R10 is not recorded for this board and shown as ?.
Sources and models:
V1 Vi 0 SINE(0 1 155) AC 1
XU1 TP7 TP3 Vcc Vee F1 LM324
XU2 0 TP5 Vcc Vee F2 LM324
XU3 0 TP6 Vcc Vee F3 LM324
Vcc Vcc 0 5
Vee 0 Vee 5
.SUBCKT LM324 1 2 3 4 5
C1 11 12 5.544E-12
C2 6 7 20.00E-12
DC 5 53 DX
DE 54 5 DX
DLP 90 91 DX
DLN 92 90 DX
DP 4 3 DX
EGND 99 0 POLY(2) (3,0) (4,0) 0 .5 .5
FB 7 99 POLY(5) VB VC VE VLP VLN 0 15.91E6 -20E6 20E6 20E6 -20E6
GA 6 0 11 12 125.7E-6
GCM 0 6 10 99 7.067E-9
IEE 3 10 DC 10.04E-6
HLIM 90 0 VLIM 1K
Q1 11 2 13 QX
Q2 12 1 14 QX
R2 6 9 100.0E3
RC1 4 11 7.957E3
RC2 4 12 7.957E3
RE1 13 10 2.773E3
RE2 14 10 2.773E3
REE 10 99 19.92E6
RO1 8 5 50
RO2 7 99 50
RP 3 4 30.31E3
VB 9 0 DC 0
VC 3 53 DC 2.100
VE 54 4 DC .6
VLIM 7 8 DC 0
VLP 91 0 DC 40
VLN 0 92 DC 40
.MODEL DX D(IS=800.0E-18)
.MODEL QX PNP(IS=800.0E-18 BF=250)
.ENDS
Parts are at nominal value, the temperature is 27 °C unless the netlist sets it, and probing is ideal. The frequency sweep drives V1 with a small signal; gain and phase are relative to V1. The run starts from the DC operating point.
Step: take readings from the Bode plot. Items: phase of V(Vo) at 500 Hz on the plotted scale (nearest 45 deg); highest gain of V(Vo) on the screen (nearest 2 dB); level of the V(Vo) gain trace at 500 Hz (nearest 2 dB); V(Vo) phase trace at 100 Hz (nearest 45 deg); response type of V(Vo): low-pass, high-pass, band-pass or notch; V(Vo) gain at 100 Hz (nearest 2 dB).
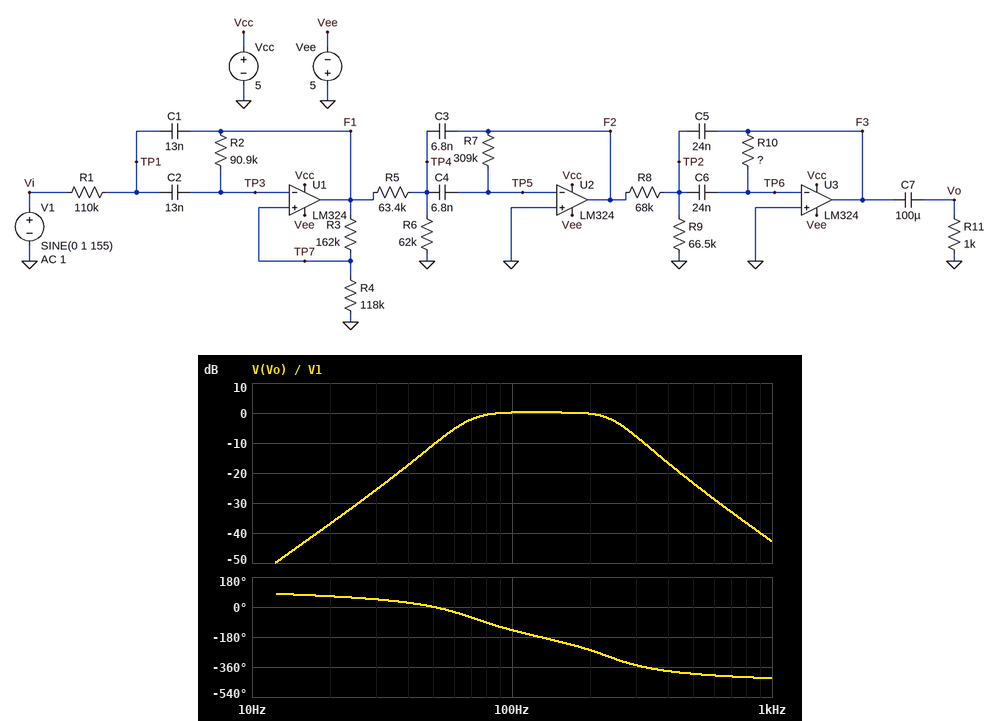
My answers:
-405 deg
0 dB
-24 dB
-135 deg
band-pass
0 dB
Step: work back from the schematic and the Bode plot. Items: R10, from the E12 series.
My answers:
270 kΩ
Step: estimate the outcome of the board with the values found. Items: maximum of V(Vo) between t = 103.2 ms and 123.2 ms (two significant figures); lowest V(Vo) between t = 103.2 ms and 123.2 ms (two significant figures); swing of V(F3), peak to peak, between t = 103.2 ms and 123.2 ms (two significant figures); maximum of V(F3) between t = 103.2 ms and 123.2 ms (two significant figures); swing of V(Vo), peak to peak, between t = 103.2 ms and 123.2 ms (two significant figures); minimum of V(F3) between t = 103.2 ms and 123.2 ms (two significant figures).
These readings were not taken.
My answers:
1.0 V
-1.0 V
2.0 V
1.0 V
2.0 V
-1.0 V
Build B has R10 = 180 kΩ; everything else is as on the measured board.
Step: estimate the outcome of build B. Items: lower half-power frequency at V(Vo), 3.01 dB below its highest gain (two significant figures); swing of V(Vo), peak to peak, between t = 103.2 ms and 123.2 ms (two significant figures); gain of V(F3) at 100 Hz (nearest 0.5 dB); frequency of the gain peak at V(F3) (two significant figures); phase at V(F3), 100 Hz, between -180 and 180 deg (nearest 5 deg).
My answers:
84 Hz
2.1 V
-0.5 dB
150 Hz
-115 deg
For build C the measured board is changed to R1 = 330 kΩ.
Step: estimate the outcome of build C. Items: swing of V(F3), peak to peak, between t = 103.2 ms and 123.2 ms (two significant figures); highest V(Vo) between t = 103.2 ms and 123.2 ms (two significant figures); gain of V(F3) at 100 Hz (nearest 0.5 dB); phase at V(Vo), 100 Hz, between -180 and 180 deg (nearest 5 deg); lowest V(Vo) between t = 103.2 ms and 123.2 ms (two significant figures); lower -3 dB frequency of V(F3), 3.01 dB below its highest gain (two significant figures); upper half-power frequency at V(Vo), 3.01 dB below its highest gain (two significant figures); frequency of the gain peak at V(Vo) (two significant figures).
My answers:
490 mV
250 mV
-11.5 dB
-165 deg
-250 mV
60 Hz
250 Hz
83 Hz
